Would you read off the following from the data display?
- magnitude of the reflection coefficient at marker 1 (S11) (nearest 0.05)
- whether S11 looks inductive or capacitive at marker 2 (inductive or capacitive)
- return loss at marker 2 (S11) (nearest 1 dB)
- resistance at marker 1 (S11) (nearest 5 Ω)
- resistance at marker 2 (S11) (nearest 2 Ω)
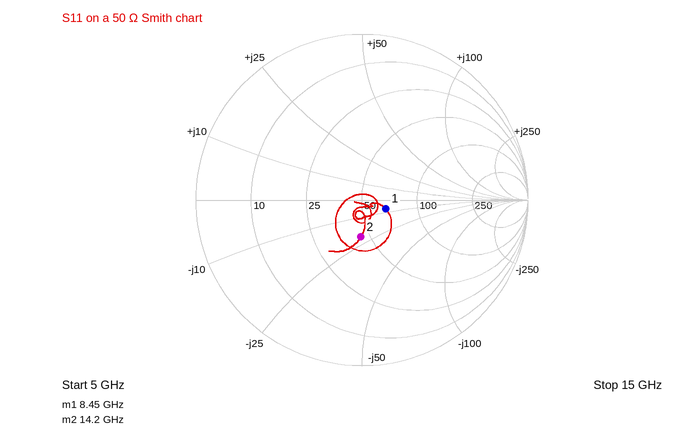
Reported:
0.15
capacitive
13 dB
65 Ω
44 Ω
